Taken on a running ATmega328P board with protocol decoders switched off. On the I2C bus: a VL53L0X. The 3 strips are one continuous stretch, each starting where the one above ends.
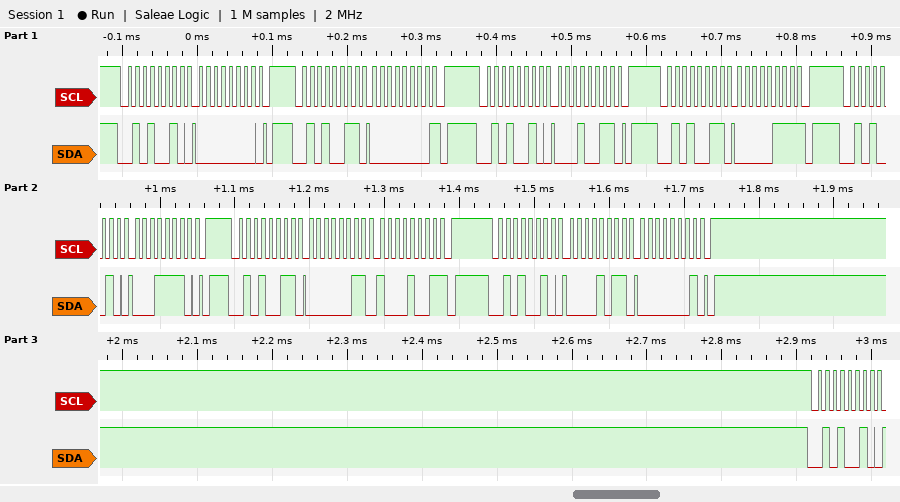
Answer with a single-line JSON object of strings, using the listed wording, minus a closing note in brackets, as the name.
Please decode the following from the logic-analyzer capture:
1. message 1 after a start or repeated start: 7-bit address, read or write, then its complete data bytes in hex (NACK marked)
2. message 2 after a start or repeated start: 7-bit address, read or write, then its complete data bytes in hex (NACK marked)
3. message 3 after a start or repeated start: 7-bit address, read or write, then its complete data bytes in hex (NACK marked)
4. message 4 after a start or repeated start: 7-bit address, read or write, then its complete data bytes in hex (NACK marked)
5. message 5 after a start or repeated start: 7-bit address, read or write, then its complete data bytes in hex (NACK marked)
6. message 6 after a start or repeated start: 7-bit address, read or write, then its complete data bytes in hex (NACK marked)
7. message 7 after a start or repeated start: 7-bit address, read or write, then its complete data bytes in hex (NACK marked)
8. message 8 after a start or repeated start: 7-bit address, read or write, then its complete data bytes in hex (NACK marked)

{"message 1 after a start or repeated start: 7-bit address, read or write, then its complete data bytes in hex": "0x29 write: 00", "message 2 after a start or repeated start: 7-bit address, read or write, then its complete data bytes in hex": "0x29 read: 00 NACK", "message 3 after a start or repeated start: 7-bit address, read or write, then its complete data bytes in hex": "0x29 write: 13", "message 4 after a start or repeated start: 7-bit address, read or write, then its complete data bytes in hex": "0x29 read: 07 NACK", "message 5 after a start or repeated start: 7-bit address, read or write, then its complete data bytes in hex": "0x29 write: 1E", "message 6 after a start or repeated start: 7-bit address, read or write, then its complete data bytes in hex": "0x29 read: 03 89 NACK", "message 7 after a start or repeated start: 7-bit address, read or write, then its complete data bytes in hex": "0x29 write: 0B 01", "message 8 after a start or repeated start: 7-bit address, read or write, then its complete data bytes in hex": "0x29 write"}
